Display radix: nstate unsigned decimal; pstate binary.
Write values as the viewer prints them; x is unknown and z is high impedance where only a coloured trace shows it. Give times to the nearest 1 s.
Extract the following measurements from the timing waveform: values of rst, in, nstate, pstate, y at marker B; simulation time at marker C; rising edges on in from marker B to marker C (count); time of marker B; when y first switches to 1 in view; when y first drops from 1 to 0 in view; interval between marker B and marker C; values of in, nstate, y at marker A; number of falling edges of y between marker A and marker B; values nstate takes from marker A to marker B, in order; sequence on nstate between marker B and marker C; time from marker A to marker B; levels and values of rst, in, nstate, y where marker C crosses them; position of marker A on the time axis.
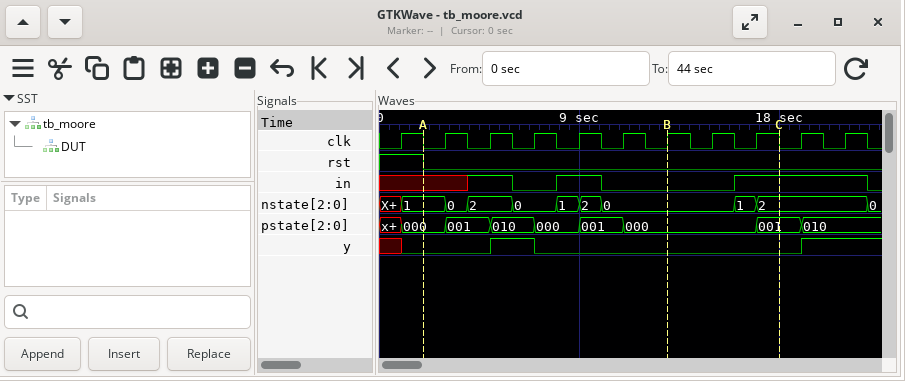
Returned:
rst=0, in=0, nstate=0, pstate=000, y=0
18 s
1
13 s
5 s
7 s
5 s
in=x, nstate=1, y=0
1
1, 0, 2, 0, 1, 2, 0
0, 1, 2
11 s
rst=0, in=1, nstate=2, y=0
2 s
